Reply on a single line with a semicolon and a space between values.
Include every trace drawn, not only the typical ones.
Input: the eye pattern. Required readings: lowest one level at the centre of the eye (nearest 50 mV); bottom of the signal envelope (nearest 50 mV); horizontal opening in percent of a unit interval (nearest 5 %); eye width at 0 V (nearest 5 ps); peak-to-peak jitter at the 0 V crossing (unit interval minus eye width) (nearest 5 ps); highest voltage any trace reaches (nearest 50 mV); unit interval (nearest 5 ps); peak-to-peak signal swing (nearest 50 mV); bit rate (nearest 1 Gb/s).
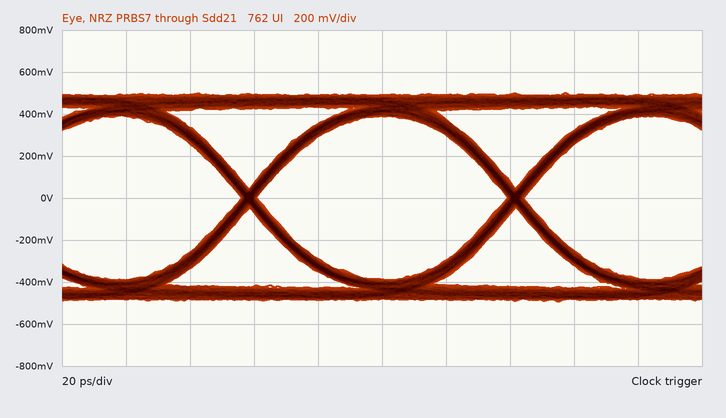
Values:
400 mV; -500 mV; 95 %; 80 ps; 5 ps; 500 mV; 85 ps; 1.00 V; 12 Gb/s
